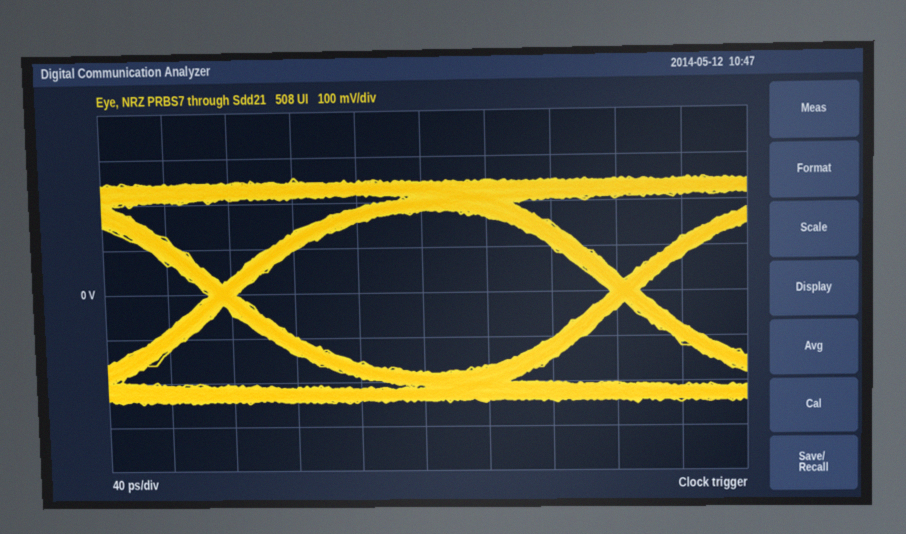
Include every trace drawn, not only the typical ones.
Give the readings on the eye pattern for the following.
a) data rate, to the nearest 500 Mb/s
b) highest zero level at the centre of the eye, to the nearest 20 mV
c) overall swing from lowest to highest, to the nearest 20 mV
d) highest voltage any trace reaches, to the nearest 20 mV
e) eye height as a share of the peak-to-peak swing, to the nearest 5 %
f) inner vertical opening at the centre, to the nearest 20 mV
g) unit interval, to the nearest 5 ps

4.0 Gb/s
-180 mV
500 mV
260 mV
70 %
360 mV
250 ps
